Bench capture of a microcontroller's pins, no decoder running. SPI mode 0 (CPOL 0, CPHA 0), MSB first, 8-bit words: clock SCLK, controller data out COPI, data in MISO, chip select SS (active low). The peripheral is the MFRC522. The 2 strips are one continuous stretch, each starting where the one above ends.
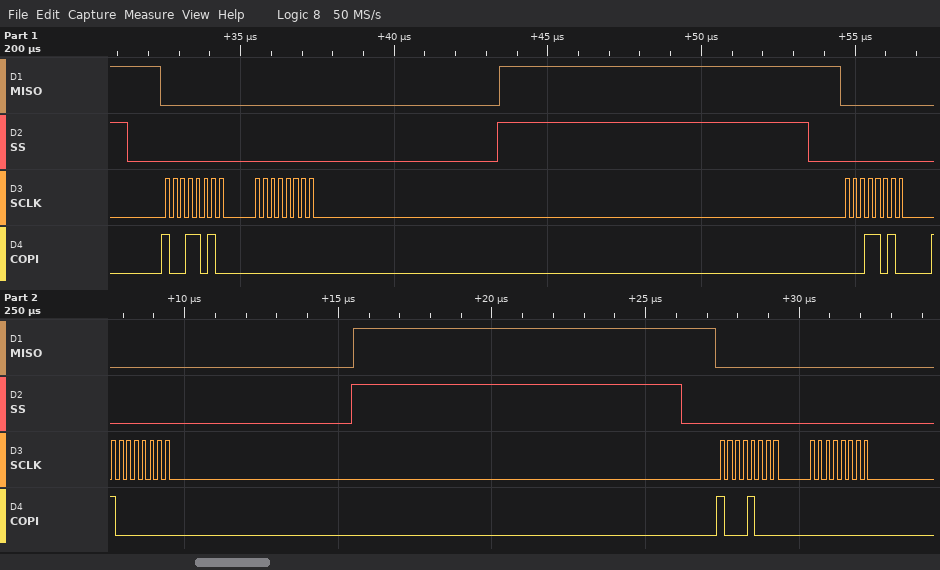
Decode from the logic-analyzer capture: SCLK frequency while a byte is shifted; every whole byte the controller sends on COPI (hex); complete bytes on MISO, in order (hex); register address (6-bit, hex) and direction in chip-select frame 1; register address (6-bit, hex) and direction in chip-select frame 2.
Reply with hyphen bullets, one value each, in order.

- 4 MHz
- 0x9A 0x00 0x1A 0x80 0x88 0x00
- 0x00 0x00 0x00 0x00 0x00 0x00
- 0x0D read
- 0x0D write
